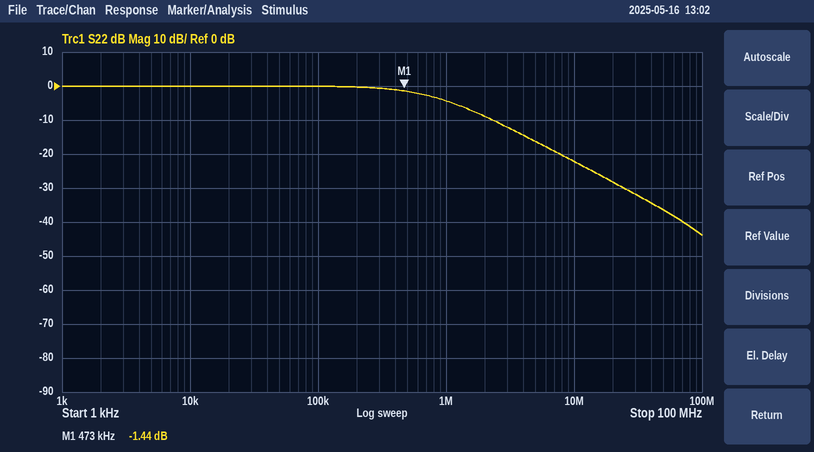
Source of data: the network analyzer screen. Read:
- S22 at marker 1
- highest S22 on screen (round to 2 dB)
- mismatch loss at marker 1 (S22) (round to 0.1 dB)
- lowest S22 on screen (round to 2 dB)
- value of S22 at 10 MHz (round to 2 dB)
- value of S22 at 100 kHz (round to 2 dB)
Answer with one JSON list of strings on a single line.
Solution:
["-1.44 dB", "0 dB", "5.5 dB", "-44 dB", "-22 dB", "0 dB"]
